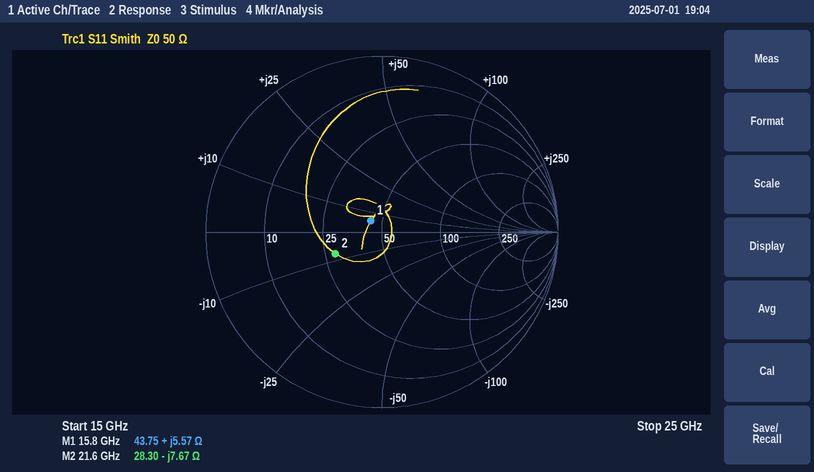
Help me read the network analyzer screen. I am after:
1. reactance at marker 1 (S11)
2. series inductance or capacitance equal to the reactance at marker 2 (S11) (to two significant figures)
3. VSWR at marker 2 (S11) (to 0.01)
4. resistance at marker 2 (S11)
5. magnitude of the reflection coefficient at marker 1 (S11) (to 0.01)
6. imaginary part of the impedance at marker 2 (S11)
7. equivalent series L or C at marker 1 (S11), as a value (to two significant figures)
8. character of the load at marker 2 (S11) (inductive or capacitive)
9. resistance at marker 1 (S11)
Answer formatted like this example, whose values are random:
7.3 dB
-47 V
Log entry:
+5.57 Ω
960 fF
1.83
28.30 Ω
0.09
-7.67 Ω
56 pH
capacitive
43.75 Ω
